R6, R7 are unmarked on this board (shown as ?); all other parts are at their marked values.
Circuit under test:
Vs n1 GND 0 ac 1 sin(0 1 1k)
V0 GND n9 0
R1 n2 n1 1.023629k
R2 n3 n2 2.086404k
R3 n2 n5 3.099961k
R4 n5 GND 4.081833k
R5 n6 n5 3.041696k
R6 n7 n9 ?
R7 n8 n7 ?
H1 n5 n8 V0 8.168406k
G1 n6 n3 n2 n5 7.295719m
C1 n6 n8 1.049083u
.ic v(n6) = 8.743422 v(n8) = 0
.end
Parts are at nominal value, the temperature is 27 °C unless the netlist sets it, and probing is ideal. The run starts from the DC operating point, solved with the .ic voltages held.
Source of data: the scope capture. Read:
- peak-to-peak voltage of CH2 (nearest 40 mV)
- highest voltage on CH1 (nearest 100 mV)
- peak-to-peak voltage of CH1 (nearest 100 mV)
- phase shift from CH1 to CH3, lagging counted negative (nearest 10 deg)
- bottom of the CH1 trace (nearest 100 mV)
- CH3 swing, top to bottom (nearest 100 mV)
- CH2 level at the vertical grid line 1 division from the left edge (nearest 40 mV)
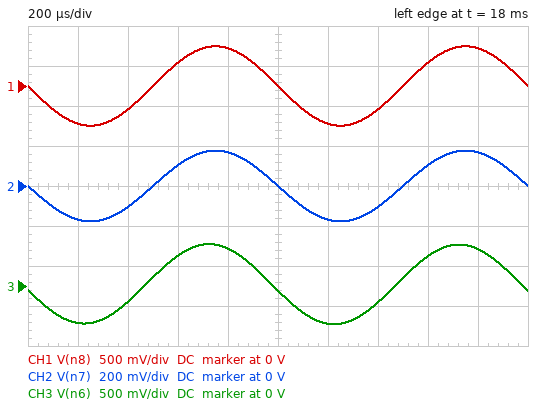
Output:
360 mV
500 mV
1.0 V
10 deg
-500 mV
1.0 V
-160 mV
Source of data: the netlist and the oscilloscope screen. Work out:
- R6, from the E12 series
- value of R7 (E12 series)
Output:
1 kΩ
1.8 kΩ
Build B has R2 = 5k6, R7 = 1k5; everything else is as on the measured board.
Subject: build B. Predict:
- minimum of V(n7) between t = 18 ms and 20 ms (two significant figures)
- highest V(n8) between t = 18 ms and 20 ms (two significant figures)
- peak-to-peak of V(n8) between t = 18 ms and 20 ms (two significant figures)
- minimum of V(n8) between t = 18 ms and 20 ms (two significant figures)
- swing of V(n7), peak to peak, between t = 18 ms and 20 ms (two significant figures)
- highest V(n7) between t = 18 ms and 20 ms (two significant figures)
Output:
-170 mV
420 mV
830 mV
-420 mV
330 mV
170 mV
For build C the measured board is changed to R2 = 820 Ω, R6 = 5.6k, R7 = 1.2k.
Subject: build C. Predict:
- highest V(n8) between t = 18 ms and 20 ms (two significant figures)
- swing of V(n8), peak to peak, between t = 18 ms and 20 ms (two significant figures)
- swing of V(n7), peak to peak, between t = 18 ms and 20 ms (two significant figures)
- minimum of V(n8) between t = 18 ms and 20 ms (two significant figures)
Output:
8.7 V
17 V
14 V
-8.7 V
